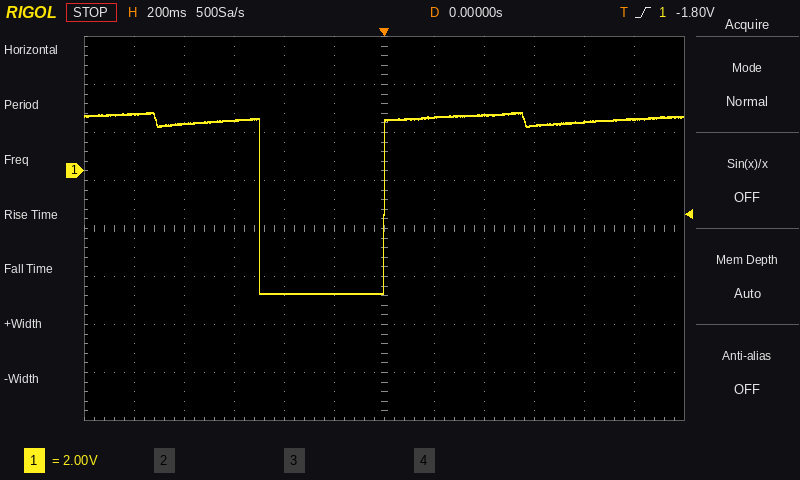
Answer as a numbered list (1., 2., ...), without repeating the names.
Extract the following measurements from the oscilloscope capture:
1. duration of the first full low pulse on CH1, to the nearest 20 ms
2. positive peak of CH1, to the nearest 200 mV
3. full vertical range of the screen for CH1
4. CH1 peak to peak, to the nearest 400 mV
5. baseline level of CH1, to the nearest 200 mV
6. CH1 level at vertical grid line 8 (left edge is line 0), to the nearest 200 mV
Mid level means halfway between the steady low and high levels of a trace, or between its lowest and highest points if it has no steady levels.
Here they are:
1. 500 ms
2. 2.4 V
3. 16 V
4. 7.6 V
5. 2.2 V
6. 2.4 V
